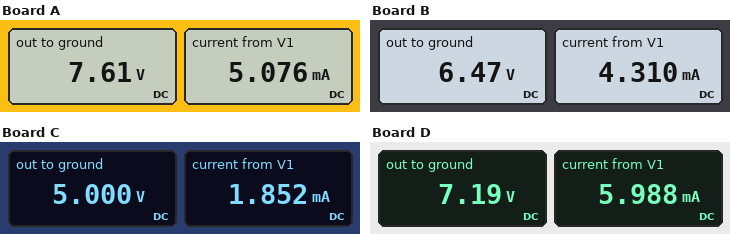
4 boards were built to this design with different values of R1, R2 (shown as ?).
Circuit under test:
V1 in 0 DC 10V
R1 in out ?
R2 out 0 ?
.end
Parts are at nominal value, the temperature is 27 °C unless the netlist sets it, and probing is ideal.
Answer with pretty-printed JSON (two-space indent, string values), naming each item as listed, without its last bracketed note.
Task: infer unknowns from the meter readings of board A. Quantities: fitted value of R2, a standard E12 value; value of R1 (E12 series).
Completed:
{
  "fitted value of R2, a standard E12 value": "1.5 kΩ",
  "value of R1": "470 Ω"
}
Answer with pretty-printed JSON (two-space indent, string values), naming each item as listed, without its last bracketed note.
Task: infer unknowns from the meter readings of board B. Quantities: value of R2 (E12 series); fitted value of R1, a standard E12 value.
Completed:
{
  "value of R2": "1.5 kΩ",
  "fitted value of R1, a standard E12 value": "820 Ω"
}
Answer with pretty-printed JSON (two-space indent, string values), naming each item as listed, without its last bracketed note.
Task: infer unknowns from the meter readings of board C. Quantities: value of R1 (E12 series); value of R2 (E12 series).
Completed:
{
  "value of R1": "2.7 kΩ",
  "value of R2": "2.7 kΩ"
}
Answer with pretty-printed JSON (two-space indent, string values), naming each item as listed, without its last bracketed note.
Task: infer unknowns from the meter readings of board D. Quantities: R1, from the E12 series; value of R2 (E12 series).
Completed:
{
  "R1, from the E12 series": "470 Ω",
  "value of R2": "1.2 kΩ"
}
